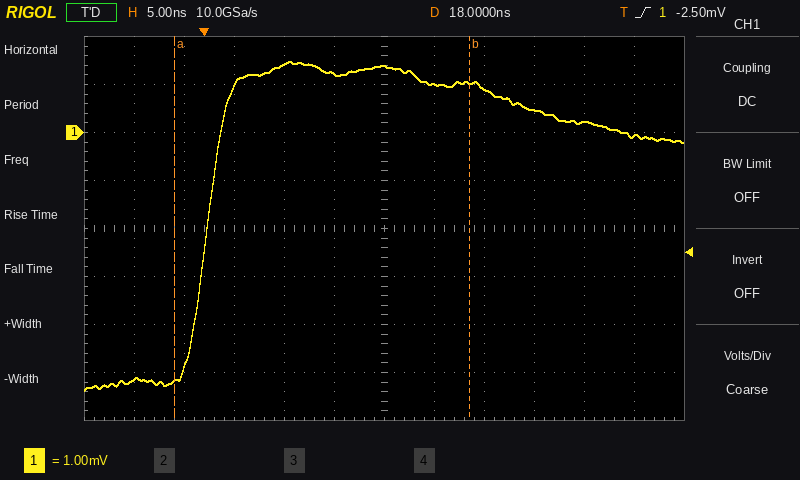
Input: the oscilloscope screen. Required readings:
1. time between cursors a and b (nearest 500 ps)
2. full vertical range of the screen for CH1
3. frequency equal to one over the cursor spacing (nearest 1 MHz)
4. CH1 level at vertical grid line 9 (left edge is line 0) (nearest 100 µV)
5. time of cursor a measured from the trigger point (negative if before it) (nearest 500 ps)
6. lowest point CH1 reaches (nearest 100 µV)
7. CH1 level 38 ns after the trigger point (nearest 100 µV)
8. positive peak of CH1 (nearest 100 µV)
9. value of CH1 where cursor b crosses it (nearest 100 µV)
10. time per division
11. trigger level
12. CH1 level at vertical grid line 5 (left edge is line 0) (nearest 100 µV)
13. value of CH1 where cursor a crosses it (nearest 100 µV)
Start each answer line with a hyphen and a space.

- 29.5 ns
- 8 mV
- 34 MHz
- 500 µV
- -3.0 ns
- -5.4 mV
- 200 µV
- 1.5 mV
- 1.0 mV
- 5 ns
- -2.50 mV
- 1.2 mV
- -5.2 mV
